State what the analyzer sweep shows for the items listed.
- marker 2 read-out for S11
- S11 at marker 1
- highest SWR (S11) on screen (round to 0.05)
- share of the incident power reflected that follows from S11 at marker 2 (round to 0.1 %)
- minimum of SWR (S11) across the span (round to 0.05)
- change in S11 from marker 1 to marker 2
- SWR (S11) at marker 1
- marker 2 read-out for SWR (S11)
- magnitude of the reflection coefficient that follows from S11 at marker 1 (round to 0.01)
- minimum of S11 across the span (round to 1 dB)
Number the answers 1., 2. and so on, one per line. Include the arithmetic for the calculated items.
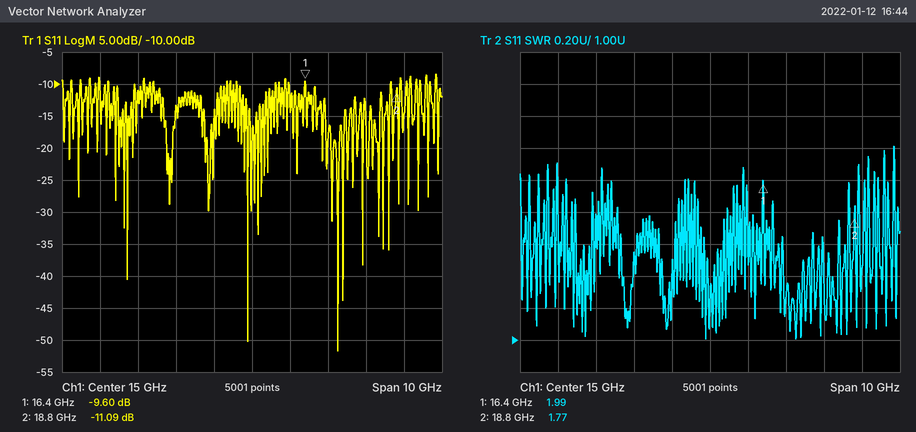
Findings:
1. -11.09 dB
2. -9.60 dB
3. 2.20
4. 10^(-11.09/10) ≈ 7.8 %
5. 1.00
6. -11.09 − (-9.6) = -1.49 dB
7. 1.99
8. 1.77
9. 10^(-9.6/20) ≈ 0.33
10. -52 dB
